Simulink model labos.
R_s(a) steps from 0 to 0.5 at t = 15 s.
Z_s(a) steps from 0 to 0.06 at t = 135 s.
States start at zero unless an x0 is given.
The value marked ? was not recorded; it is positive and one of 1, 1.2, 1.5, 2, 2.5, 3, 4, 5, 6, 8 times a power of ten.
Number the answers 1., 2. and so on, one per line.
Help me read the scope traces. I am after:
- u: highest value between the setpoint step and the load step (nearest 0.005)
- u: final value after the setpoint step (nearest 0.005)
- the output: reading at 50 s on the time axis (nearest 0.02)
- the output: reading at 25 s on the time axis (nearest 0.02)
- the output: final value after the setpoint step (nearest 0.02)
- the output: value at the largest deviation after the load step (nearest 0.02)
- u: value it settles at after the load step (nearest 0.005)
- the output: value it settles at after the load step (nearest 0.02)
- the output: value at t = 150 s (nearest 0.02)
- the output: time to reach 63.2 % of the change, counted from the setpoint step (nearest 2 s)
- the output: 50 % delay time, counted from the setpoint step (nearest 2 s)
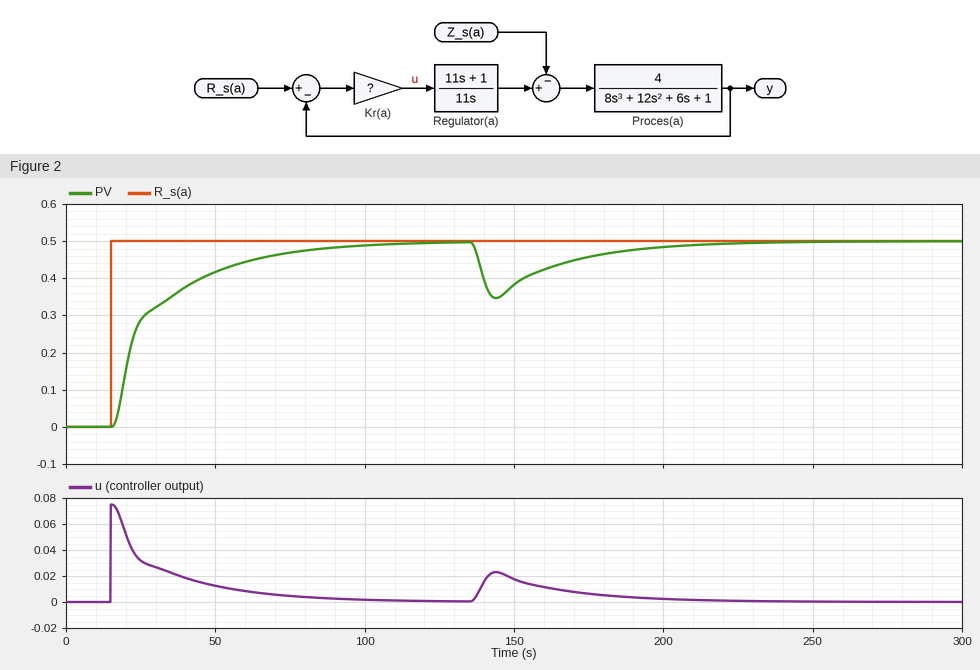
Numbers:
1. 0.075
2. 0.000
3. 0.42
4. 0.28
5. 0.50
6. 0.34
7. 0.000
8. 0.50
9. 0.38
10. 14 s
11. 8 s
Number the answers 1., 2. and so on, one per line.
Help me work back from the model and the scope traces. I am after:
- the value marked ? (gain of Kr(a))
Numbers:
1. 0.15
